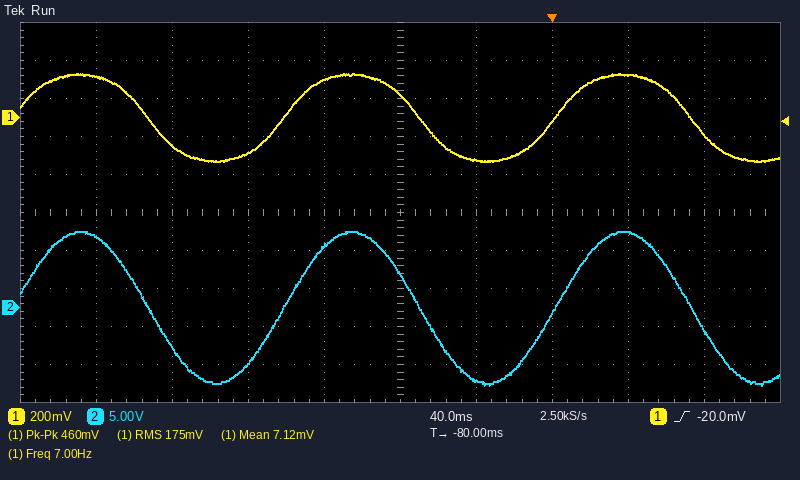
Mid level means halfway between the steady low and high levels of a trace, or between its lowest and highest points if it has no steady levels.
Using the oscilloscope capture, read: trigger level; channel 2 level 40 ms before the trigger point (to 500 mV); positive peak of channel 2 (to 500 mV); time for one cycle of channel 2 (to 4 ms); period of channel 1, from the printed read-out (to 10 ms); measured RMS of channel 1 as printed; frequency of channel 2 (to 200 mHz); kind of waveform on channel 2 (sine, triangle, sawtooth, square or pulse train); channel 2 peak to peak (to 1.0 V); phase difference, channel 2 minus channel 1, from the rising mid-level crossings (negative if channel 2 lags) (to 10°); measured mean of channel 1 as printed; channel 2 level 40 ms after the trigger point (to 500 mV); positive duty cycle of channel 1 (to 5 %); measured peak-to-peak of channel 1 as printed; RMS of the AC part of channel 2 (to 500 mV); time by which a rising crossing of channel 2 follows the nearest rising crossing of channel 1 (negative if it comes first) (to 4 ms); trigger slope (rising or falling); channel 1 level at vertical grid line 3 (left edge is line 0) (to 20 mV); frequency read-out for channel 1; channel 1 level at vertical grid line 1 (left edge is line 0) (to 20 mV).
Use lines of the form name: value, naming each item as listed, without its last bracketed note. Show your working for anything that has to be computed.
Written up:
trigger level: -20.0 mV
channel 2 level 40 ms before the trigger point: -9.5 V
positive peak of channel 2: 10.0 V
time for one cycle of channel 2: 144 ms
period of channel 1, from the printed read-out: 1 / 7.00 Hz ≈ 143 ms, so 140 ms to the nearest 10 ms
measured RMS of channel 1 as printed: 175 mV
frequency of channel 2: 1 / 144 ms ≈ 6.94 Hz, so 7.0 Hz to the nearest 200 mHz
kind of waveform on channel 2: sine
channel 2 peak to peak: 20.0 V
phase difference, channel 2 minus channel 1, from the rising mid-level crossings (negative if channel 2 lags): −360° × (0 ms) / 144 ms ≈ 0°
measured mean of channel 1 as printed: 7.12 mV
channel 2 level 40 ms after the trigger point: 10.0 V
positive duty cycle of channel 1: 50 %
measured peak-to-peak of channel 1 as printed: 460 mV
RMS of the AC part of channel 2: 20.0 V / (2√2) ≈ 7.07 V, so 7.0 V to the nearest 500 mV
time by which a rising crossing of channel 2 follows the nearest rising crossing of channel 1 (negative if it comes first): 0 ms
trigger slope: rising
channel 1 level at vertical grid line 3 (left edge is line 0): -180 mV
frequency read-out for channel 1: 7.00 Hz
channel 1 level at vertical grid line 1 (left edge is line 0): 220 mV
